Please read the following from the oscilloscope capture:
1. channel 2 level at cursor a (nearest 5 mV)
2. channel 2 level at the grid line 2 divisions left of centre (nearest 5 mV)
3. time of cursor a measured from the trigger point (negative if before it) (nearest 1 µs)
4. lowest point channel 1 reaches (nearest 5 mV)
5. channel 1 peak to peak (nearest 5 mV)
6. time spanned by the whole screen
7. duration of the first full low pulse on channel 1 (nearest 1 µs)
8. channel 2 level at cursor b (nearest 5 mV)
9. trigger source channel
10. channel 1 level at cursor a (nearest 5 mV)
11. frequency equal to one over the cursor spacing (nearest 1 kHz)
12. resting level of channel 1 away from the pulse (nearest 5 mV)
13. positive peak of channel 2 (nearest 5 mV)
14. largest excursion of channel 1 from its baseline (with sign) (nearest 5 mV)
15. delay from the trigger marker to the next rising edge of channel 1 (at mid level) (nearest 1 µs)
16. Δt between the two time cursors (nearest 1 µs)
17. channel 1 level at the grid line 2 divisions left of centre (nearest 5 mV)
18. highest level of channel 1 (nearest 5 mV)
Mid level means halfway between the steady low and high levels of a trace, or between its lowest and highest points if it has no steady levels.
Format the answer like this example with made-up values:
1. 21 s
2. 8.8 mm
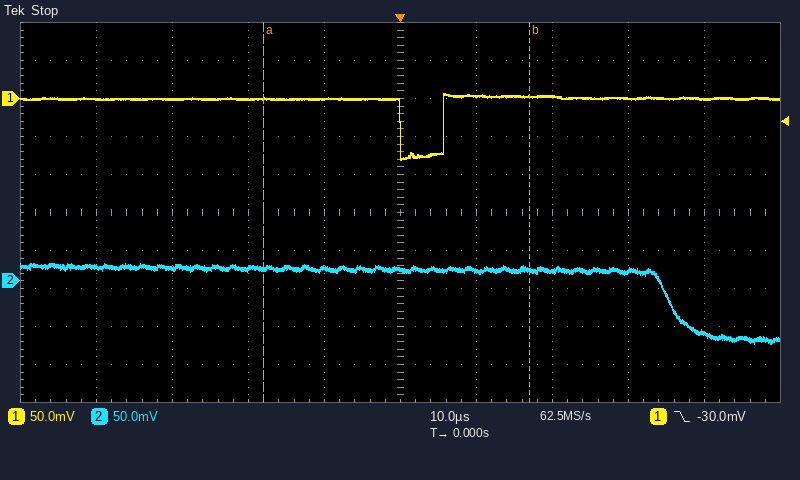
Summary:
1. 15 mV
2. 15 mV
3. -18 µs
4. -80 mV
5. 85 mV
6. 100 µs
7. 6 µs
8. 15 mV
9. channel 1
10. 0 mV
11. 29 kHz
12. 0 mV
13. 25 mV
14. -80 mV
15. 6 µs
16. 35 µs
17. 0 mV
18. 5 mV
